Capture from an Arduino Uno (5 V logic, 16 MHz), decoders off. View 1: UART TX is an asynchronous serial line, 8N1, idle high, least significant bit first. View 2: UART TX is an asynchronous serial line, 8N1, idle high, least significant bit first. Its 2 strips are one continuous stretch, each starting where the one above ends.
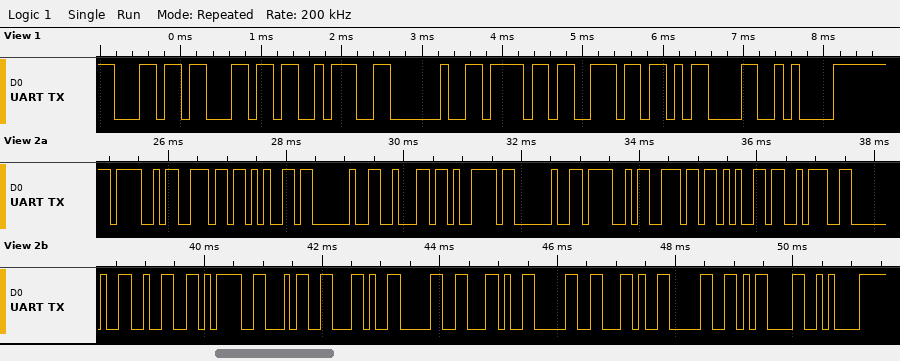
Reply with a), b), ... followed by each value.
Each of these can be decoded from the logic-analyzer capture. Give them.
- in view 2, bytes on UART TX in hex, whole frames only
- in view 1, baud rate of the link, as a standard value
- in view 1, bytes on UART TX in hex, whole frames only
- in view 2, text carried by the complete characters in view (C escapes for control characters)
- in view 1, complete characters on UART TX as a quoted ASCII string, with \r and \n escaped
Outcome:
a) 4F 6E 65 20 62 79 20 4F 6E 65 3A 20 32 3D 34 2C 30 2C 30 2C 30 0D 0A
b) 9600 baud
c) 0x6C 0x6C 0x3A 0x20 0x6F 0x6E 0x0D 0x0A
d) "One by One: 2=4,0,0,0\r\n"
e) "ll: on\r\n"
